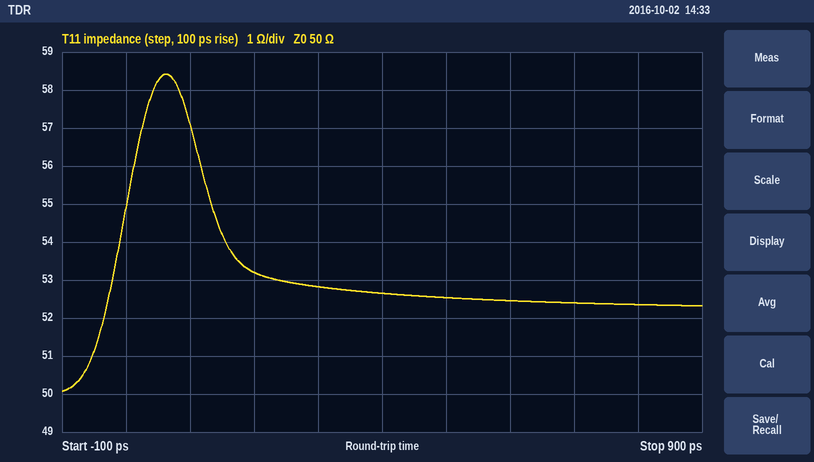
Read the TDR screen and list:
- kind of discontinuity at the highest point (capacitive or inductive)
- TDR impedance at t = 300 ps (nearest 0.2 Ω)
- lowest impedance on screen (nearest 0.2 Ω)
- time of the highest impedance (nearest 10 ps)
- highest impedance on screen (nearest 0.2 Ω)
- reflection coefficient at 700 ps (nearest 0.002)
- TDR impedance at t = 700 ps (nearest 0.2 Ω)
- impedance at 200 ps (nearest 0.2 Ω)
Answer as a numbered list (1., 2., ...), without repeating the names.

1. inductive
2. 52.8 Ω
3. 50.0 Ω
4. 60 ps
5. 58.4 Ω
6. +0.024
7. 52.4 Ω
8. 53.2 Ω
